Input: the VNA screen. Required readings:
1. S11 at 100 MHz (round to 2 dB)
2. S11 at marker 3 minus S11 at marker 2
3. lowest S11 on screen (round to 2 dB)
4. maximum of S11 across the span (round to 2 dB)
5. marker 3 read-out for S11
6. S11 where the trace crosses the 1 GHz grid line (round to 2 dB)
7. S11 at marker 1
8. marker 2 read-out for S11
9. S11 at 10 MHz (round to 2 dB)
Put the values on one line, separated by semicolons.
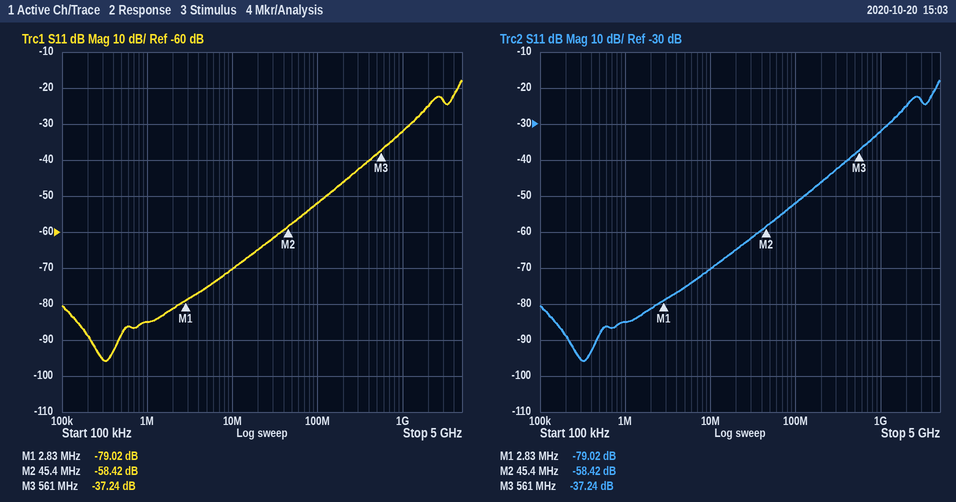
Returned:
-52 dB; 21.18 dB; -96 dB; -18 dB; -37.24 dB; -32 dB; -79.02 dB; -58.42 dB; -70 dB
